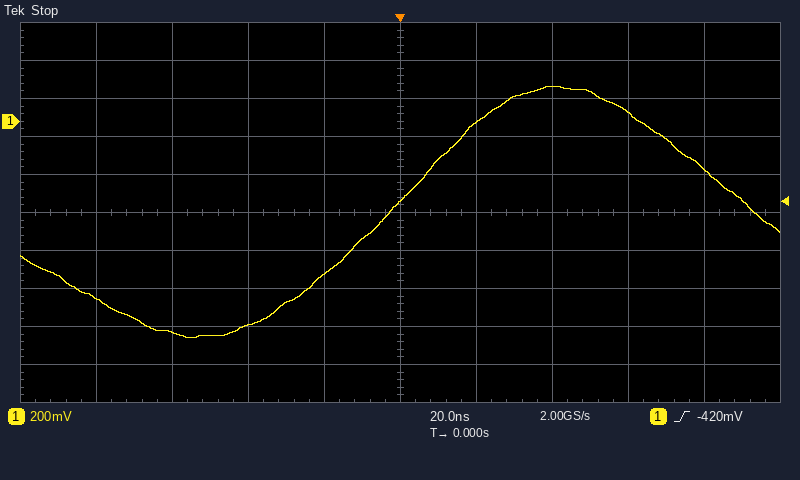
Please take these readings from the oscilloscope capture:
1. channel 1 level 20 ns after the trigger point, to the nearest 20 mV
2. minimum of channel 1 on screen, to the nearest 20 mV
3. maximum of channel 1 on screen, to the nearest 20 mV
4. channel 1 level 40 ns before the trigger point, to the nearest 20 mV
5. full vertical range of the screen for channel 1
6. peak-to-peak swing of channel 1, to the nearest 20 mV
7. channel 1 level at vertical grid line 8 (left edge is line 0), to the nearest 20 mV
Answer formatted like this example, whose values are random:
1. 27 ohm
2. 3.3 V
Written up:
1. 0 mV
2. -1.14 V
3. 180 mV
4. -1.08 V
5. 2 V
6. 1.32 V
7. 40 mV
